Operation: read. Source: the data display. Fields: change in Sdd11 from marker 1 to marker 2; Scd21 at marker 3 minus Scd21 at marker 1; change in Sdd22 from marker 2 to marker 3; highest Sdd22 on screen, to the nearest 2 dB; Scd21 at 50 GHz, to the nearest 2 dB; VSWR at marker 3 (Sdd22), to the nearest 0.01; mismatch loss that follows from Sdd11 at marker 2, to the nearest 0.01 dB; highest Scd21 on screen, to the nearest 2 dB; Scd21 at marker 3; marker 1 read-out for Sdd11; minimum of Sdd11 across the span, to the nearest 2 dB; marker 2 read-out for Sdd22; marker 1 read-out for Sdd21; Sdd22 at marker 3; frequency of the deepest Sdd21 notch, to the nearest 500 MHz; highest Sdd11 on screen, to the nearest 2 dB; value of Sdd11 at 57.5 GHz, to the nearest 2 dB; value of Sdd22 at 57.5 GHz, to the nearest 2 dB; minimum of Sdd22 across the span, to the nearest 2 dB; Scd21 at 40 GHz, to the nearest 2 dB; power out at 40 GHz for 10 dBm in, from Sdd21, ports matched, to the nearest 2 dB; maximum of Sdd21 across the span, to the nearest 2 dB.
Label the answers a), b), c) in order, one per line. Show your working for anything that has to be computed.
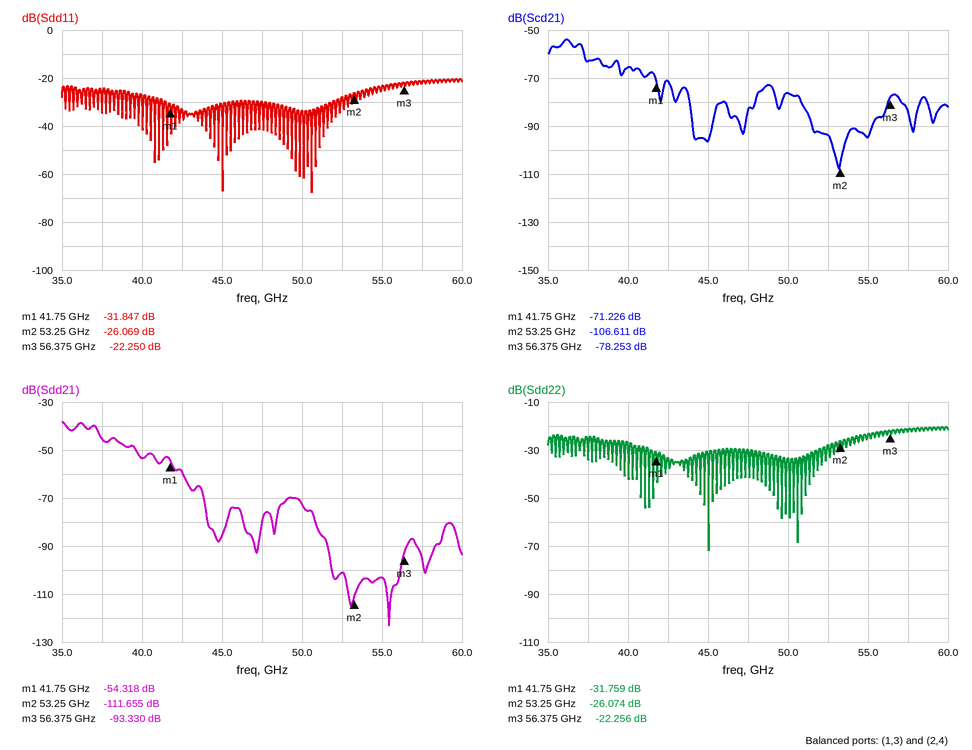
a) -26.069 − (-31.847) = 5.778 dB
b) -78.253 − (-71.226) = -7.027 dB
c) -22.256 − (-26.074) = 3.818 dB
d) -20 dB
e) -76 dB
f) (1 + 0.0771)/(1 − 0.0771) ≈ 1.17
g) −10 log10(1 − 10^(-26.069/10)) ≈ 0.01 dB
h) -54 dB
i) -78.253 dB
j) -31.847 dB
k) -68 dB
l) -26.074 dB
m) -54.318 dB
n) -22.256 dB
o) 55.5 GHz
p) -20 dB
q) -22 dB
r) -22 dB
s) -72 dB
t) -66 dB
u) 10 dBm + (-54 dB) = -44 dBm
v) -38 dB
